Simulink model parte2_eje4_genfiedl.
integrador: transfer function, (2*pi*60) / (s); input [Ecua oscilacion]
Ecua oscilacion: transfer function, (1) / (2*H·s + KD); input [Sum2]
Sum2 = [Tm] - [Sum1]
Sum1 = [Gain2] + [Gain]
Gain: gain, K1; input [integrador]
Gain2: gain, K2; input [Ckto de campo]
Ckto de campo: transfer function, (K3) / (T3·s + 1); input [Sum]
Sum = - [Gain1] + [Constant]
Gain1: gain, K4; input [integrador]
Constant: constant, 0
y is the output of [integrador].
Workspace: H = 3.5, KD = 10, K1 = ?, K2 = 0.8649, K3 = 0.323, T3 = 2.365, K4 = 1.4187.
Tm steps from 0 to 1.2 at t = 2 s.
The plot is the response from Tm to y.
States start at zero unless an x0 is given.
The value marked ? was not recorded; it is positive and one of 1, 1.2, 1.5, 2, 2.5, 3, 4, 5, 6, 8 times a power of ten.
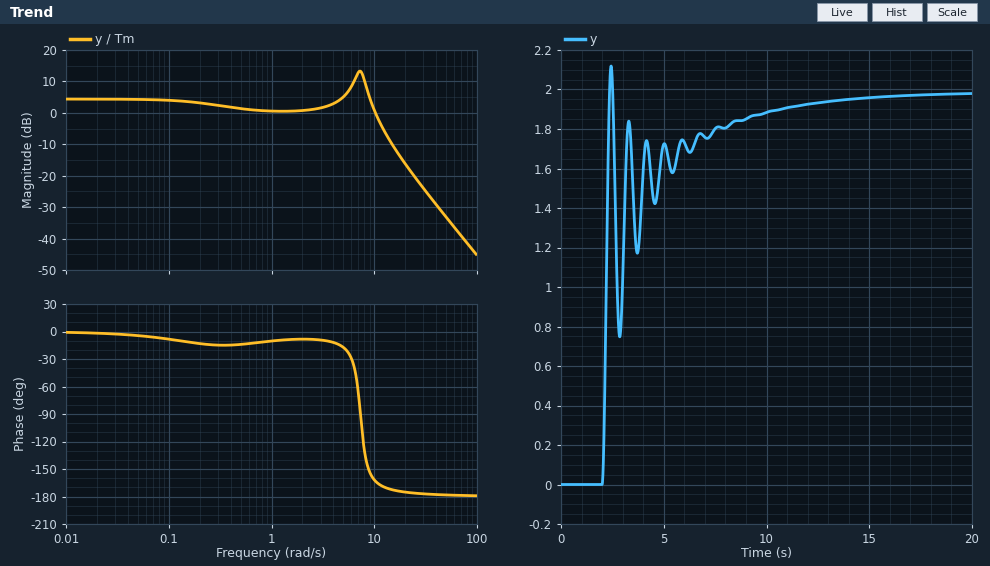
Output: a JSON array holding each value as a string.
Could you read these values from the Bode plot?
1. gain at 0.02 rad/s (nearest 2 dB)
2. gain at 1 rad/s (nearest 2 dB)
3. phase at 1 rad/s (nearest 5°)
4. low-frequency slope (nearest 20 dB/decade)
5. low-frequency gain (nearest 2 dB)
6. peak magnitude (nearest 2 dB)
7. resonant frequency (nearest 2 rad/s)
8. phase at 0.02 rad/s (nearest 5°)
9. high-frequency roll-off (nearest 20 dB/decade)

["4 dB", "0 dB", "-10°", "0 dB/decade", "4 dB", "14 dB", "8 rad/s", "0°", "-40 dB/decade"]
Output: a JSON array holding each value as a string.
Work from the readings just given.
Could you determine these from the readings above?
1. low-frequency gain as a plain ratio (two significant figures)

["1.6"]
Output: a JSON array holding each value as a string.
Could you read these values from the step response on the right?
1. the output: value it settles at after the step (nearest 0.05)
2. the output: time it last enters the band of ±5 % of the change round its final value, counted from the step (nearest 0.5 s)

["2.00", "8.0 s"]
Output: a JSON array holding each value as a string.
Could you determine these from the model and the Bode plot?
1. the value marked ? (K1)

["1"]
